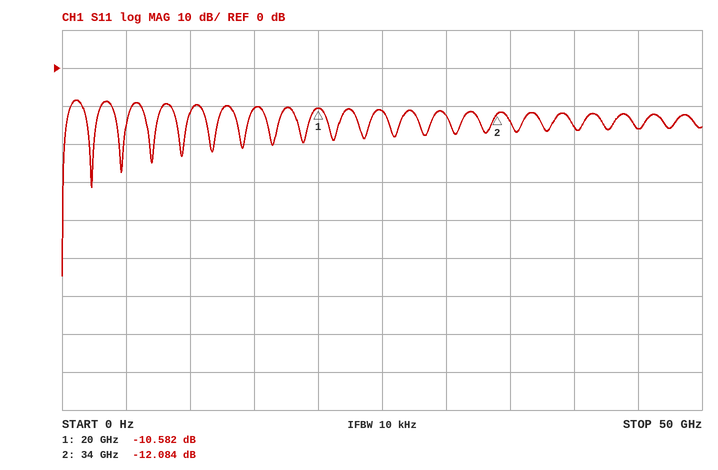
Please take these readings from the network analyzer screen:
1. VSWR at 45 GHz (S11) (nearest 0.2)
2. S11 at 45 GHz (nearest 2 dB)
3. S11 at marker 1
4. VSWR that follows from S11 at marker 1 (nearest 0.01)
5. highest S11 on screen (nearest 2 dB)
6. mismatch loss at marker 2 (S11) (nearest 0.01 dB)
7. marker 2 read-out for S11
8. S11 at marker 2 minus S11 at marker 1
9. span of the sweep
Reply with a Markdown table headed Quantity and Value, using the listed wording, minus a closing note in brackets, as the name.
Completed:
| Quantity | Value |
|---|---|
| VSWR at 45 GHz (S11) | 1.4 |
| S11 at 45 GHz | -16 dB |
| S11 at marker 1 | -10.582 dB |
| VSWR that follows from S11 at marker 1 | 1.84 |
| highest S11 on screen | -8 dB |
| mismatch loss at marker 2 (S11) | 0.28 dB |
| marker 2 read-out for S11 | -12.084 dB |
| S11 at marker 2 minus S11 at marker 1 | -1.502 dB |
| span of the sweep | 50 GHz |
